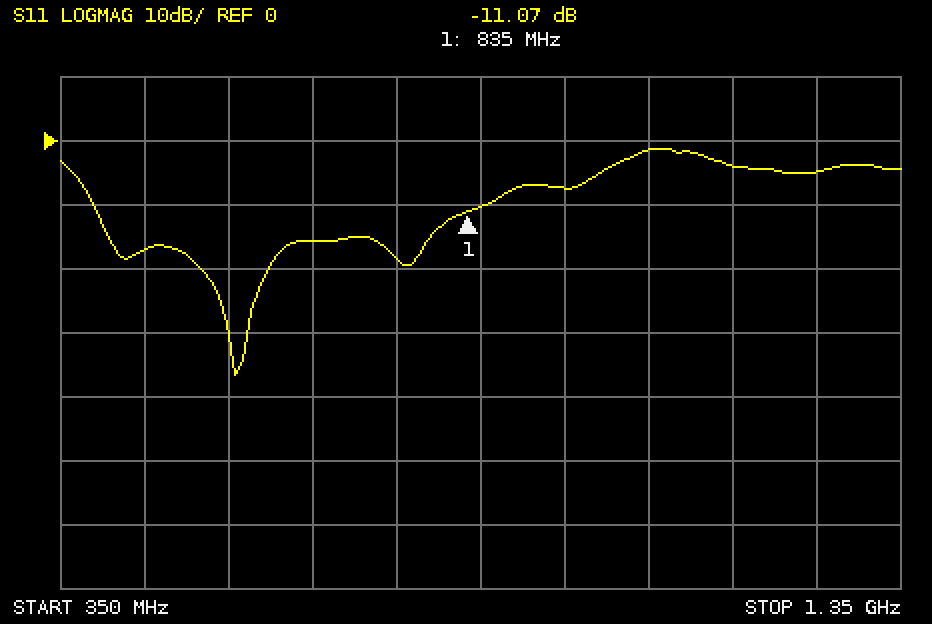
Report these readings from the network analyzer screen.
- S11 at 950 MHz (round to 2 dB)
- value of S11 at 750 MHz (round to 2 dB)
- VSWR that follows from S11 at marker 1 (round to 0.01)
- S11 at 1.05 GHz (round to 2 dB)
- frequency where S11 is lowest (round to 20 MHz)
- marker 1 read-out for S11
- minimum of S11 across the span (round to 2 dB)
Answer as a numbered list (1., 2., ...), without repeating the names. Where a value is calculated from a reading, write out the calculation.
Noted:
1. -8 dB
2. -18 dB
3. (1 + 0.2796)/(1 − 0.2796) ≈ 1.78
4. -2 dB
5. 560 MHz
6. -11.07 dB
7. -36 dB
